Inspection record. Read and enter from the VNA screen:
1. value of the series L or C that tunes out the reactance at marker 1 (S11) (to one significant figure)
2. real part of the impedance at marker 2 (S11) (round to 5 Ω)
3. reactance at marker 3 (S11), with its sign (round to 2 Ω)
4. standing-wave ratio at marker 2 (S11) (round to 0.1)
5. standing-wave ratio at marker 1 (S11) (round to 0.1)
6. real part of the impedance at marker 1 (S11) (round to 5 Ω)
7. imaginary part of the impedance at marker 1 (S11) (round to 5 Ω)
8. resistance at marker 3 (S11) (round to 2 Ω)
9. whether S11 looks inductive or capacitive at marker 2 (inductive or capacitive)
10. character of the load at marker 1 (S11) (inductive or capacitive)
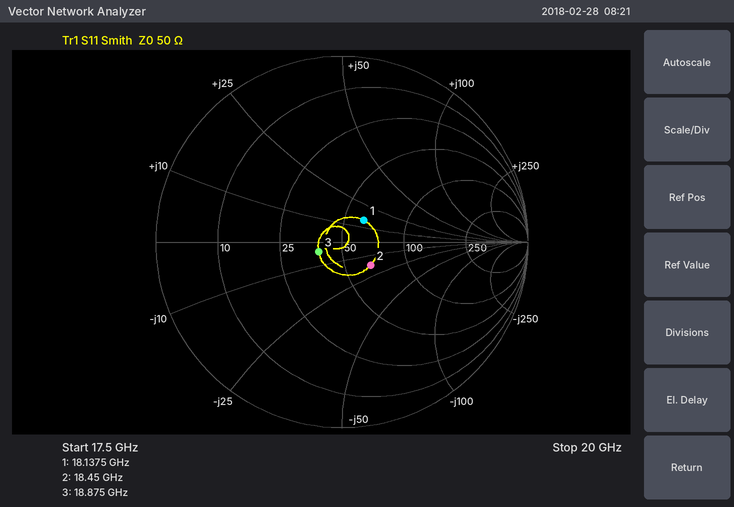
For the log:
600 fF
65 Ω
-4 Ω
1.5
1.4
60 Ω
+15 Ω
38 Ω
capacitive
inductive
